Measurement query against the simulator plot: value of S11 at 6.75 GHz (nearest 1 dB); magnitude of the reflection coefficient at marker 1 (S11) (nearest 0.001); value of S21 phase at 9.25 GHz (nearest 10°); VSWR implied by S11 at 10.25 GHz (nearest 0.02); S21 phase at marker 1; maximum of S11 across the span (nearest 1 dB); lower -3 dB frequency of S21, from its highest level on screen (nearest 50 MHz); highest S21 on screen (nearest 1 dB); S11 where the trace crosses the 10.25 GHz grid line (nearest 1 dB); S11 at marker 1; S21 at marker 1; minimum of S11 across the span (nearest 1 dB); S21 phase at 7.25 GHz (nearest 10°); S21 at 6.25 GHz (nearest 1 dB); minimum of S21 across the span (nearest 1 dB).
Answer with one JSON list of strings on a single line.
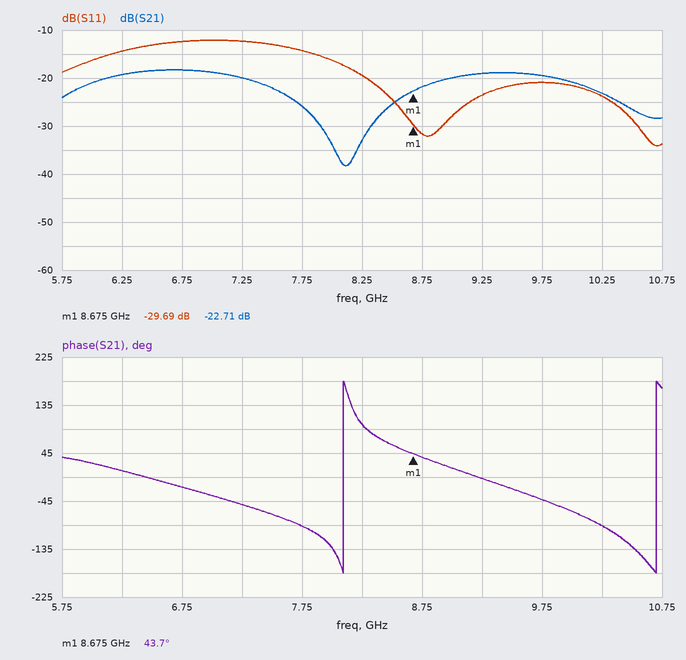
["-12 dB", "0.033", "0°", "1.14", "43.7°", "-12 dB", "5.95 GHz", "-18 dB", "-24 dB", "-29.69 dB", "-22.71 dB", "-34 dB", "-50°", "-19 dB", "-38 dB"]
